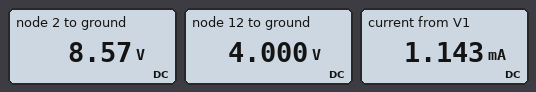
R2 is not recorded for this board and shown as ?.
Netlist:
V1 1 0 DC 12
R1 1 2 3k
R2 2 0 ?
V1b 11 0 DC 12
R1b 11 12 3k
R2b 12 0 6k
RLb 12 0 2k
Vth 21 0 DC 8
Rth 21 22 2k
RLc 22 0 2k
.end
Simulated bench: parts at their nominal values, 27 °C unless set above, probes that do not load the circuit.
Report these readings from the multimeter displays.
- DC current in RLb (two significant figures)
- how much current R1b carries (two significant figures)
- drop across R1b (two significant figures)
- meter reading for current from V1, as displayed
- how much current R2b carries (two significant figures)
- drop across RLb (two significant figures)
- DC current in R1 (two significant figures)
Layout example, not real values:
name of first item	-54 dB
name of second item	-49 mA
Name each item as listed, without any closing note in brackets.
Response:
DC current in RLb	2.0 mA
how much current R1b carries	2.7 mA
drop across R1b	8.0 V
meter reading for current from V1, as displayed	1.143 mA
how much current R2b carries	670 µA
drop across RLb	4.0 V
DC current in R1	1.1 mA
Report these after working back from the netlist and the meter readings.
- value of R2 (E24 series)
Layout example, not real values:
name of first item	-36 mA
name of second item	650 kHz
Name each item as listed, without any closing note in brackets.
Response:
value of R2	7.5 kΩ
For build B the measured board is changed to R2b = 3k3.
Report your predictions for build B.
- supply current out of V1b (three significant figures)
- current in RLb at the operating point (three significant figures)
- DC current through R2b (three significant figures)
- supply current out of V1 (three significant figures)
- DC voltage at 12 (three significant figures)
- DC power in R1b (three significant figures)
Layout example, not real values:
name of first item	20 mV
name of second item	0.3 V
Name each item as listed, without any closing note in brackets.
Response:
supply current out of V1b	2.83 mA
current in RLb at the operating point	1.76 mA
DC current through R2b	1.07 mA
supply current out of V1	1.14 mA
DC voltage at 12	3.52 V
DC power in R1b	24.0 mW
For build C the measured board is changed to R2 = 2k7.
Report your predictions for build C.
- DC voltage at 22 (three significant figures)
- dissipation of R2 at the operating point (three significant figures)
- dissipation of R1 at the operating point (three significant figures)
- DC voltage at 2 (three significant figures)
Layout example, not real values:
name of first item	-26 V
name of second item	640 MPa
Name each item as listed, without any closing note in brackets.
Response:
DC voltage at 22	4.00 V
dissipation of R2 at the operating point	12.0 mW
dissipation of R1 at the operating point	13.3 mW
DC voltage at 2	5.68 V
